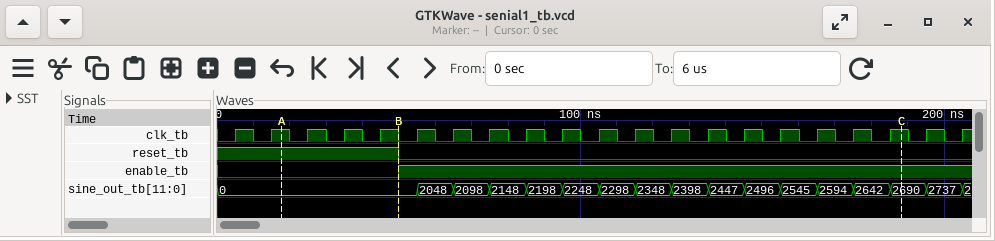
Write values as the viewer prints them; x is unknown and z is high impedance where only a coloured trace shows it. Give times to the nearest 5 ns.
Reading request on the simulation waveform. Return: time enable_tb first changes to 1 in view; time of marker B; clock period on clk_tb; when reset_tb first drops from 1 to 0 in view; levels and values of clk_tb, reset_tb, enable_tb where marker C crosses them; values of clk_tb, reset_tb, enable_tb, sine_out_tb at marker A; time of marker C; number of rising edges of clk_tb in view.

50 ns
50 ns
10 ns
50 ns
clk_tb=1, reset_tb=0, enable_tb=1
clk_tb=1, reset_tb=1, enable_tb=0, sine_out_tb=0
190 ns
21
